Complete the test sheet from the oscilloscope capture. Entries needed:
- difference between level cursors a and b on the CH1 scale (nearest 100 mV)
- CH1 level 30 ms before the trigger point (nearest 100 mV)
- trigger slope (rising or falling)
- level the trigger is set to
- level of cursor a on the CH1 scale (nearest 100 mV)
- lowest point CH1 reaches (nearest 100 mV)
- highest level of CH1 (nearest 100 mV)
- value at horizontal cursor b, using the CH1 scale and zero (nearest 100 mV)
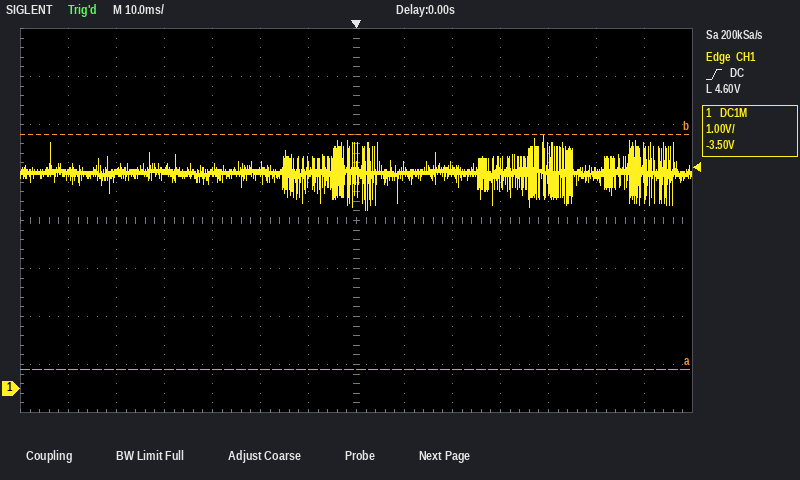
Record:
4.9 V
4.5 V
rising
4.60 V
400 mV
3.7 V
5.3 V
5.3 V
